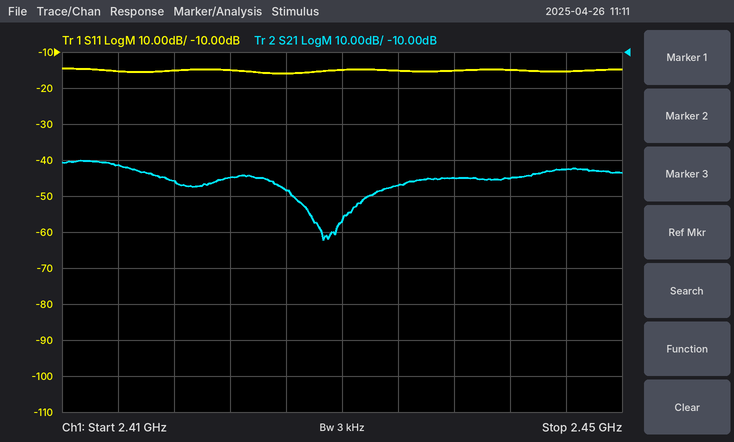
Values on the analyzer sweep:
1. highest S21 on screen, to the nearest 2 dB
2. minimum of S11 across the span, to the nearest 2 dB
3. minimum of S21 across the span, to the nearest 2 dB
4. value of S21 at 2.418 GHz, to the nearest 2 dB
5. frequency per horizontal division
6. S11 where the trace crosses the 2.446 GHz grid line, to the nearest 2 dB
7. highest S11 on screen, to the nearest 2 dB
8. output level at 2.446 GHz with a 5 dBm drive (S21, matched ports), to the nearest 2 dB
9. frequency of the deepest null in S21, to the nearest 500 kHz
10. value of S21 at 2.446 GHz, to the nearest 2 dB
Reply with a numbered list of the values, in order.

1. -40 dB
2. -16 dB
3. -62 dB
4. -46 dB
5. 4 MHz
6. -16 dB
7. -14 dB
8. -38 dBm
9. 2.4285 GHz
10. -42 dB
